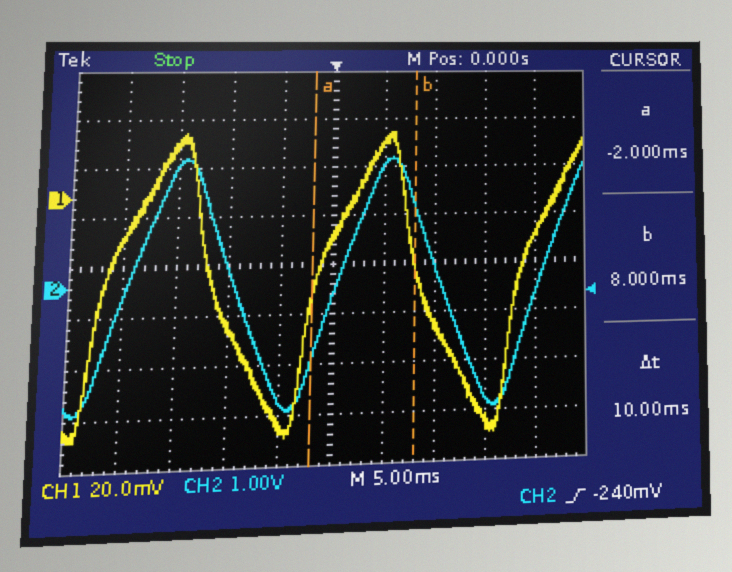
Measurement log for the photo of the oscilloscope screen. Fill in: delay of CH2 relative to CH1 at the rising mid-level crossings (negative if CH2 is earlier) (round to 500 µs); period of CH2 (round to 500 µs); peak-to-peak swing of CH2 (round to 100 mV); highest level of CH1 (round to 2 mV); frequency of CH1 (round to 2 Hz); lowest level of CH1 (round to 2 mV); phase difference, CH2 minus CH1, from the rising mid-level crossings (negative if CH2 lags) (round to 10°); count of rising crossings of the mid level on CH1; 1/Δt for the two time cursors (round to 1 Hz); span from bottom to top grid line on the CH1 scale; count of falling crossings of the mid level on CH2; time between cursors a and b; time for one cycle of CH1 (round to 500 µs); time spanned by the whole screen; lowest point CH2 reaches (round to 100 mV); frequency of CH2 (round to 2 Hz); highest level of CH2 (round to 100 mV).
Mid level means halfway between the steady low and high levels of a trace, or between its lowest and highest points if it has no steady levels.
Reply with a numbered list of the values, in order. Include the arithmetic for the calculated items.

1. +2.0 ms
2. 20.0 ms
3. 2.6 V − (-2.5 V) = 5.1 V
4. 26 mV
5. 1 / 20.0 ms ≈ 50 Hz
6. -96 mV
7. −360° × (+2.0 ms) / 20.0 ms ≈ -36.0°, so -40° to the nearest 10°
8. 3
9. 1 / 10 ms ≈ 100 Hz
10. 160 mV
11. 2
12. 10 ms
13. 20.0 ms
14. 50 ms
15. -2.5 V
16. 1 / 20.0 ms ≈ 50 Hz
17. 2.6 V
